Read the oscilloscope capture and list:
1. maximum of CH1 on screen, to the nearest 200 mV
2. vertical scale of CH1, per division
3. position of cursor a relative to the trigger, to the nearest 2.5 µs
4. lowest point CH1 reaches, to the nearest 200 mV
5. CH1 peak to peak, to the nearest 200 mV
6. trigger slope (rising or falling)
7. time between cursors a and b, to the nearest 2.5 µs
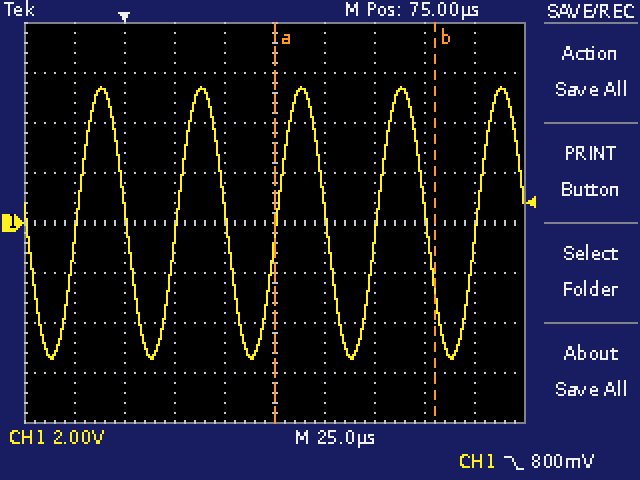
5.4 V
2 V
+75.0 µs
-5.4 V
10.8 V
falling
80.0 µs
